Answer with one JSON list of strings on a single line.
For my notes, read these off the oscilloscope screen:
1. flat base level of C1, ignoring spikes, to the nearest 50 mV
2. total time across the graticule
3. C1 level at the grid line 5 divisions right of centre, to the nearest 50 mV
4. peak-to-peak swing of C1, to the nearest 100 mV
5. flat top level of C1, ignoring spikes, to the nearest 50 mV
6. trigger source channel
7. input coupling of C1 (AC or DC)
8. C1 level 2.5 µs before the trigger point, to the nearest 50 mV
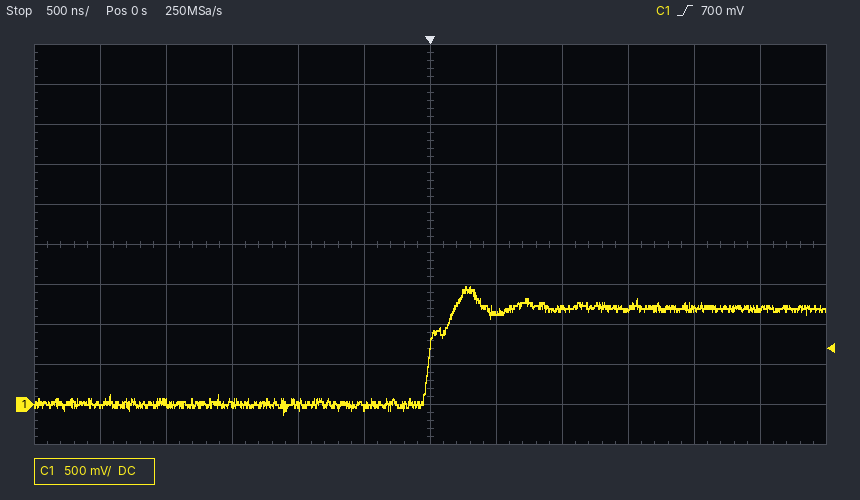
["0 mV", "6 µs", "1.20 V", "1.60 V", "1.20 V", "C1", "DC", "0 mV"]
